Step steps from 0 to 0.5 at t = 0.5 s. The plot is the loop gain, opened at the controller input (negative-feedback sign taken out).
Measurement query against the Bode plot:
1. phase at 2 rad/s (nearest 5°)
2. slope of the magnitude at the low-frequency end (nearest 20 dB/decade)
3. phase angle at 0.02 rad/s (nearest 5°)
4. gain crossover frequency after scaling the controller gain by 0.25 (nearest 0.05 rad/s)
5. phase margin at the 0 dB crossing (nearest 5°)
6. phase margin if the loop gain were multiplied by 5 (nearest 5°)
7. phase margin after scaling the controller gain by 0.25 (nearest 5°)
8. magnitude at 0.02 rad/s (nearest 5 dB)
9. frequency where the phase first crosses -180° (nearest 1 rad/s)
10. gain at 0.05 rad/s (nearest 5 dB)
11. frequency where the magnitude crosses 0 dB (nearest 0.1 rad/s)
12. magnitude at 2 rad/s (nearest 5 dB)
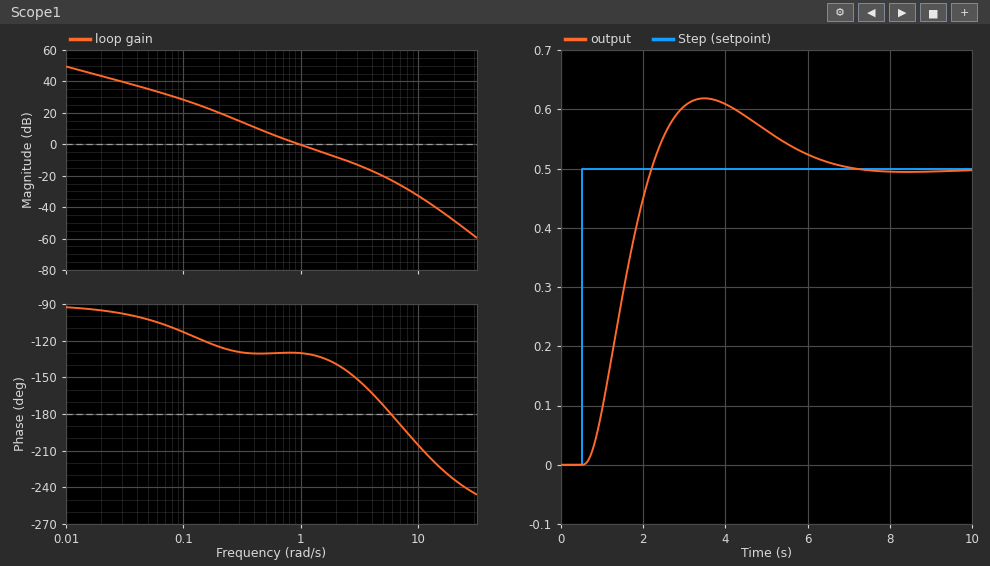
-140°
-20 dB/decade
-95°
0.35 rad/s
50°
25°
50°
45 dB
6 rad/s
35 dB
1.0 rad/s
-10 dB
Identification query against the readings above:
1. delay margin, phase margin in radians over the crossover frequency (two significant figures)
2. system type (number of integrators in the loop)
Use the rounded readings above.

0.87 s
1
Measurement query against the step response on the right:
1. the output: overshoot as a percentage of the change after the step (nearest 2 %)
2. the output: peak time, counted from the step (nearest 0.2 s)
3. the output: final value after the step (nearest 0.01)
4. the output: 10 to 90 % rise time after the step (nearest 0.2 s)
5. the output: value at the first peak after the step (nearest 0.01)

24 %
3.0 s
0.50
1.2 s
0.62
